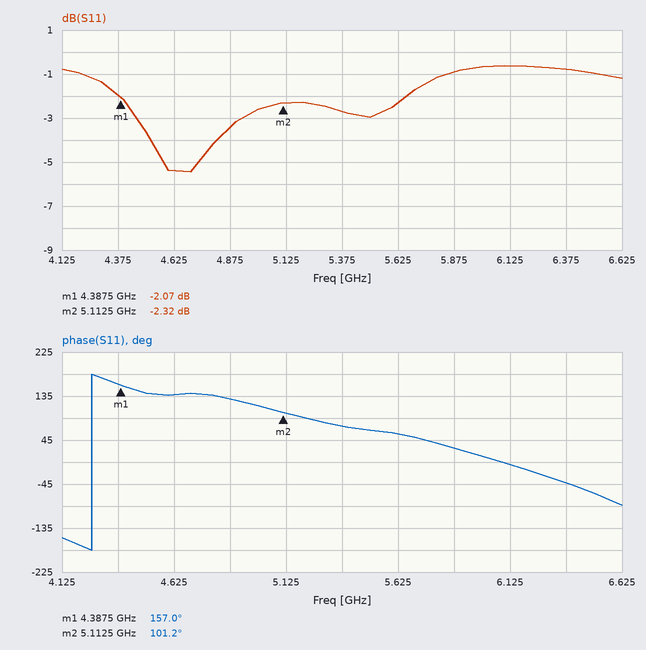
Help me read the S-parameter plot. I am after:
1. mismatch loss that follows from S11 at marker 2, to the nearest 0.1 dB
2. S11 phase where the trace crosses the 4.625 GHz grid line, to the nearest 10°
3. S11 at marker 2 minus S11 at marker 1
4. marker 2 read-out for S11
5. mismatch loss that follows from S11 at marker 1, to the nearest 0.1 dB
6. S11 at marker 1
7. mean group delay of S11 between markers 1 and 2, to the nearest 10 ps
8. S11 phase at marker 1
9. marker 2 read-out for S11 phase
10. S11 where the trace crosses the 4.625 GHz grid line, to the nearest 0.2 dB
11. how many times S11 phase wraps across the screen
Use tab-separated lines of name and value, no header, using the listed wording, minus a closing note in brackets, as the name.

mismatch loss that follows from S11 at marker 2, to the nearest 0.1 dB	3.8 dB
S11 phase where the trace crosses the 4.625 GHz grid line, to the nearest 10°	140°
S11 at marker 2 minus S11 at marker 1	-0.25 dB
marker 2 read-out for S11	-2.32 dB
mismatch loss that follows from S11 at marker 1, to the nearest 0.1 dB	4.2 dB
S11 at marker 1	-2.07 dB
mean group delay of S11 between markers 1 and 2, to the nearest 10 ps	210 ps
S11 phase at marker 1	157.0°
marker 2 read-out for S11 phase	101.2°
S11 where the trace crosses the 4.625 GHz grid line, to the nearest 0.2 dB	-5.4 dB
how many times S11 phase wraps across the screen	1
